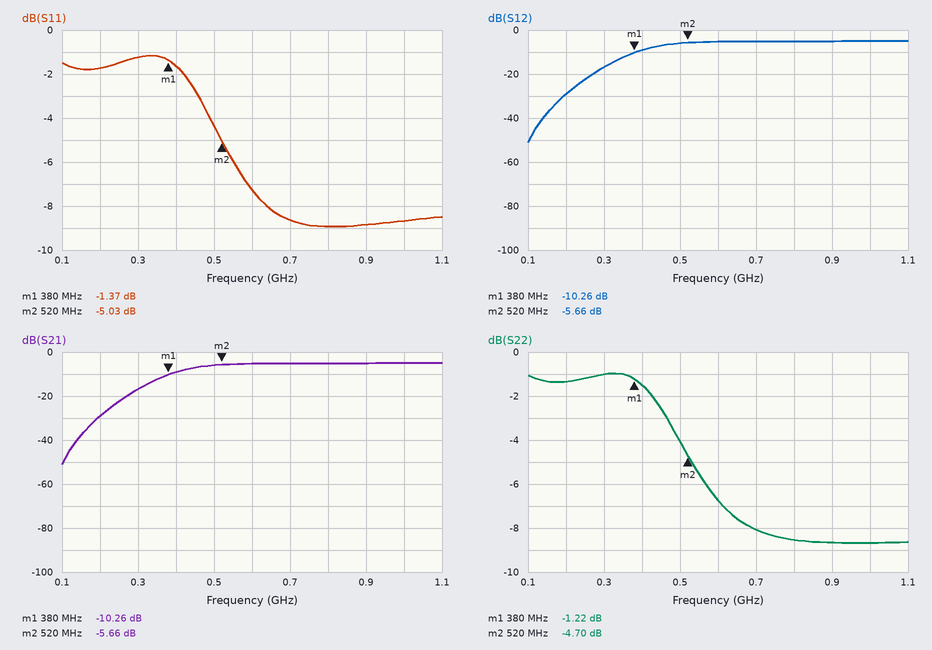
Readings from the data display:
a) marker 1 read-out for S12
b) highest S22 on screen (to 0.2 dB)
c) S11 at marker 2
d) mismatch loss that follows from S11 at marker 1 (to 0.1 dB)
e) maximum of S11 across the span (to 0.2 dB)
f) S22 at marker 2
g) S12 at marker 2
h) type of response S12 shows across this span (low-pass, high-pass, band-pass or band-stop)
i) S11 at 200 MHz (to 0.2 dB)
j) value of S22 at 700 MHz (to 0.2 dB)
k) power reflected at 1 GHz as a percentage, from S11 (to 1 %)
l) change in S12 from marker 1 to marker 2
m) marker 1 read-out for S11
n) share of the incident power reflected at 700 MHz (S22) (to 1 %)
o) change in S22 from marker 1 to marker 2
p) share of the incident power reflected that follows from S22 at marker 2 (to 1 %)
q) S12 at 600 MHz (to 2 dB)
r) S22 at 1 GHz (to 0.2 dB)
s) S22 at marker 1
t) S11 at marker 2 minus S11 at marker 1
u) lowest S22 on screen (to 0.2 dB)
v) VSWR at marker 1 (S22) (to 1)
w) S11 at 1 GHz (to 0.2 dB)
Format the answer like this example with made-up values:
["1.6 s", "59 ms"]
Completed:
["-10.26 dB", "-1.0 dB", "-5.03 dB", "5.7 dB", "-1.2 dB", "-4.70 dB", "-5.66 dB", "high-pass", "-1.8 dB", "-8.0 dB", "14 %", "4.60 dB", "-1.37 dB", "16 %", "-3.48 dB", "34 %", "-6 dB", "-8.6 dB", "-1.22 dB", "-3.66 dB", "-8.6 dB", "14", "-8.6 dB"]
